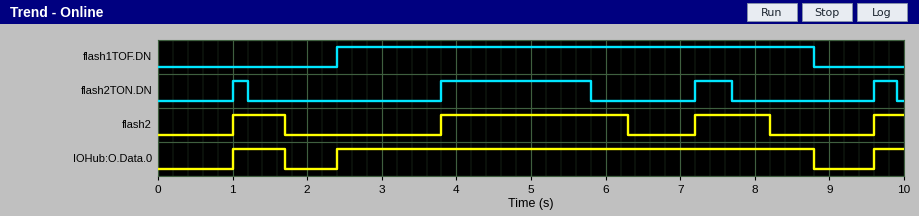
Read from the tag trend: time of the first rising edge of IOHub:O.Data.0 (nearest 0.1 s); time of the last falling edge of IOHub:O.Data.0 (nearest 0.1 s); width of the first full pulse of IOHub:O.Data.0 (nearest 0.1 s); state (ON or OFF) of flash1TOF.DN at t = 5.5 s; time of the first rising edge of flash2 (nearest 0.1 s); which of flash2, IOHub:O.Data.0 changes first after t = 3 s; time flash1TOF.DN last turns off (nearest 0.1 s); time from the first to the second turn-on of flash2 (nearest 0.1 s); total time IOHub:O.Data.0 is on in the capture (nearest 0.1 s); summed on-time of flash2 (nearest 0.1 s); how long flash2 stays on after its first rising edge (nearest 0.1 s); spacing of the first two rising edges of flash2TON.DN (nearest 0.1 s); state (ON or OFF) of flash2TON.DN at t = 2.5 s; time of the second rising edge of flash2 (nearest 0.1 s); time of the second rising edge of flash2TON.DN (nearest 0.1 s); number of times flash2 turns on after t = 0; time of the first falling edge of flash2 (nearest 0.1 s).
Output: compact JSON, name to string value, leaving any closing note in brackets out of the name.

{"time of the first rising edge of IOHub:O.Data.0": "1.0 s", "time of the last falling edge of IOHub:O.Data.0": "8.8 s", "width of the first full pulse of IOHub:O.Data.0": "0.7 s", "state (ON or OFF) of flash1TOF.DN at t = 5.5 s": "ON", "time of the first rising edge of flash2": "1.0 s", "which of flash2, IOHub:O.Data.0 changes first after t = 3 s": "flash2", "time flash1TOF.DN last turns off": "8.8 s", "time from the first to the second turn-on of flash2": "2.8 s", "total time IOHub:O.Data.0 is on in the capture": "7.5 s", "summed on-time of flash2": "4.6 s", "how long flash2 stays on after its first rising edge": "0.7 s", "spacing of the first two rising edges of flash2TON.DN": "2.8 s", "state (ON or OFF) of flash2TON.DN at t = 2.5 s": "OFF", "time of the second rising edge of flash2": "3.8 s", "time of the second rising edge of flash2TON.DN": "3.8 s", "number of times flash2 turns on after t = 0": "4", "time of the first falling edge of flash2": "1.7 s"}
